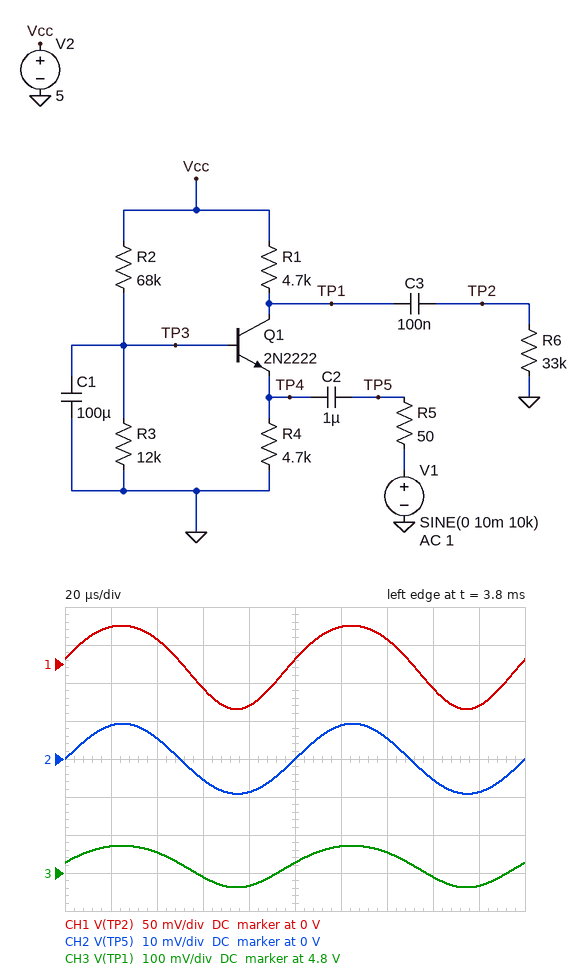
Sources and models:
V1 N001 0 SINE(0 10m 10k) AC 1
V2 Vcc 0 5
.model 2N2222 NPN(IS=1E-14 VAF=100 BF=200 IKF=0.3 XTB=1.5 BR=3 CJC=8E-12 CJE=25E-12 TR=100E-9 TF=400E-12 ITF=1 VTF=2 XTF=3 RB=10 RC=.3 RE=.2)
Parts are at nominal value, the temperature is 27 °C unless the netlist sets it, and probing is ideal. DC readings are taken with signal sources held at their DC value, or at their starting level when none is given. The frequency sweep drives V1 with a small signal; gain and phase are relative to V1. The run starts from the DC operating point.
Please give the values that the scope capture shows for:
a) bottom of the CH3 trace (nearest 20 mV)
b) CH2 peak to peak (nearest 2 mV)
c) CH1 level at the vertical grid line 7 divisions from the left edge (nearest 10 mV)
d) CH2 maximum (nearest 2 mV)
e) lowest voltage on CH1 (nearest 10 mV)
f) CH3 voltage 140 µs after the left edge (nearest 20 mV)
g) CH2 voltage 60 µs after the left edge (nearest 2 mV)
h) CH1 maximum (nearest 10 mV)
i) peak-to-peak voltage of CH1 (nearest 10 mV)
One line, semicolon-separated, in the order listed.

4.76 V; 18 mV; 30 mV; 10 mV; -60 mV; 4.86 V; -6 mV; 50 mV; 110 mV
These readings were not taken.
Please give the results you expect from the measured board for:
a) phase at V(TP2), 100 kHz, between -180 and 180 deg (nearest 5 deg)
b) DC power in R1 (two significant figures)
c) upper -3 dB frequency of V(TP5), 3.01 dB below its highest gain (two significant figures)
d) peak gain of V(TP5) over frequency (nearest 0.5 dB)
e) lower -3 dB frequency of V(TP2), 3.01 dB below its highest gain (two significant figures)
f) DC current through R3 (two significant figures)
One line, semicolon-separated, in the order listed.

0 deg; 6.7 µW; 67 MHz; 0 dB; 250 Hz; 62 µA
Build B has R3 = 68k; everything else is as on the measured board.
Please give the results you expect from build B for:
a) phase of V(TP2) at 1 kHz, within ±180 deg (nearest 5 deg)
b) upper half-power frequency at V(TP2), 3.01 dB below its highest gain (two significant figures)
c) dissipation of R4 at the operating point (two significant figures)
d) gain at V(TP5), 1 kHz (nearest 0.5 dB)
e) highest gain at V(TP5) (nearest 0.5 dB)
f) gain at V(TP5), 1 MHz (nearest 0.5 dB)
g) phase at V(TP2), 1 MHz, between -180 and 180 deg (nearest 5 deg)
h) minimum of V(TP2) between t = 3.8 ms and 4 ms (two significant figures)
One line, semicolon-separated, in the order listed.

55 deg; 5.6 MHz; 690 µW; -1.0 dB; 0 dB; -5.0 dB; -10 deg; -350 mV
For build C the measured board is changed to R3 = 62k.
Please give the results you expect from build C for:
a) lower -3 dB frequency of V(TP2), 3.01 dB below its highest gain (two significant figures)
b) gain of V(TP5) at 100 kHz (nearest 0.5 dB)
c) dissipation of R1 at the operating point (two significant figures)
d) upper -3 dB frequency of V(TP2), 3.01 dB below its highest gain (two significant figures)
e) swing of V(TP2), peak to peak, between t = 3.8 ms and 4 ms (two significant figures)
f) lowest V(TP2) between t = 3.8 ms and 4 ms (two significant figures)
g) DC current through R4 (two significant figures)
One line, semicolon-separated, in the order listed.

1.3 kHz; -4.5 dB; 610 µW; 5.9 MHz; 650 mV; -340 mV; 360 µA
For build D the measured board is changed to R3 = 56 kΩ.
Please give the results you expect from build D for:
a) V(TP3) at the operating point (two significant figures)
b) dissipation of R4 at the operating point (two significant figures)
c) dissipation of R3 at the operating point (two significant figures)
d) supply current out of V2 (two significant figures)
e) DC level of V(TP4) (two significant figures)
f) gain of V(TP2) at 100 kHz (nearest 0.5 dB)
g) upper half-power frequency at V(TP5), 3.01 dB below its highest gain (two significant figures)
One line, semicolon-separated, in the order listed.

2.2 V; 530 µW; 87 µW; 380 µA; 1.6 V; 30.0 dB; 2.4 kHz
